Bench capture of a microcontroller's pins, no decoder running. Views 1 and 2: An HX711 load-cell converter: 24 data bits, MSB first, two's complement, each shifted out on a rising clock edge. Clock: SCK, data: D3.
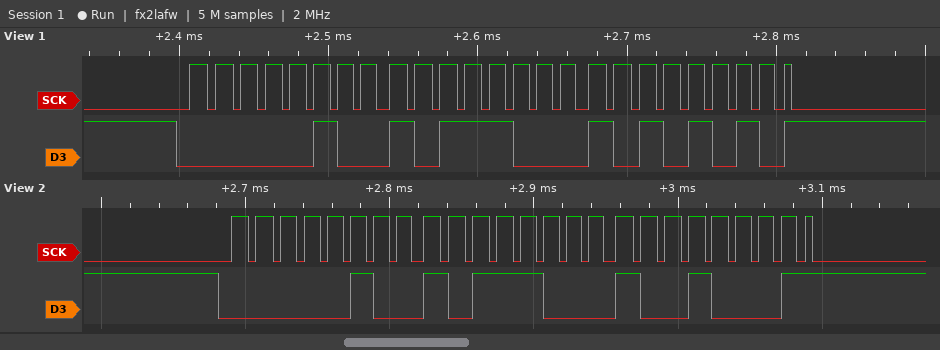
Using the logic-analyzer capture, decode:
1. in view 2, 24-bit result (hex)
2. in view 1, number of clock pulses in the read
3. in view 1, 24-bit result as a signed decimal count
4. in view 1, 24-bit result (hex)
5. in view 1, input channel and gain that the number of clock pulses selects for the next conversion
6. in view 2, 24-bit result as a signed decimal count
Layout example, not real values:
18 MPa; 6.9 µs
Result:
0x04B891; 25; 309418; 0x04B8AA; channel A, gain 128; 309393
